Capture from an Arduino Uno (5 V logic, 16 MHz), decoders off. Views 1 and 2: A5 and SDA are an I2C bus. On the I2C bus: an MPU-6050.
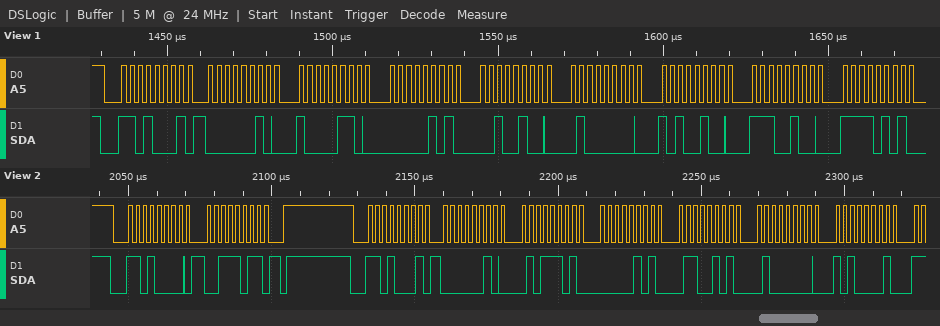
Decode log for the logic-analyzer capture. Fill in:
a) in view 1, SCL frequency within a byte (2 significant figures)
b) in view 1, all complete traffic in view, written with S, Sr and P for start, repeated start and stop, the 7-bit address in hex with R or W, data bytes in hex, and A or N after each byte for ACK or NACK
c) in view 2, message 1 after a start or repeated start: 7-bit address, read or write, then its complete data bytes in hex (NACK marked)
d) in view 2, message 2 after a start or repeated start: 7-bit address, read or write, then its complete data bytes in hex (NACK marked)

400 kHz
S 68R A 02 A 86 A 05 A 24 A 40 A A4 A E4 A F5 A
0x68 write: 3B
0x68 read: 02 5D 05 65 40 A1
